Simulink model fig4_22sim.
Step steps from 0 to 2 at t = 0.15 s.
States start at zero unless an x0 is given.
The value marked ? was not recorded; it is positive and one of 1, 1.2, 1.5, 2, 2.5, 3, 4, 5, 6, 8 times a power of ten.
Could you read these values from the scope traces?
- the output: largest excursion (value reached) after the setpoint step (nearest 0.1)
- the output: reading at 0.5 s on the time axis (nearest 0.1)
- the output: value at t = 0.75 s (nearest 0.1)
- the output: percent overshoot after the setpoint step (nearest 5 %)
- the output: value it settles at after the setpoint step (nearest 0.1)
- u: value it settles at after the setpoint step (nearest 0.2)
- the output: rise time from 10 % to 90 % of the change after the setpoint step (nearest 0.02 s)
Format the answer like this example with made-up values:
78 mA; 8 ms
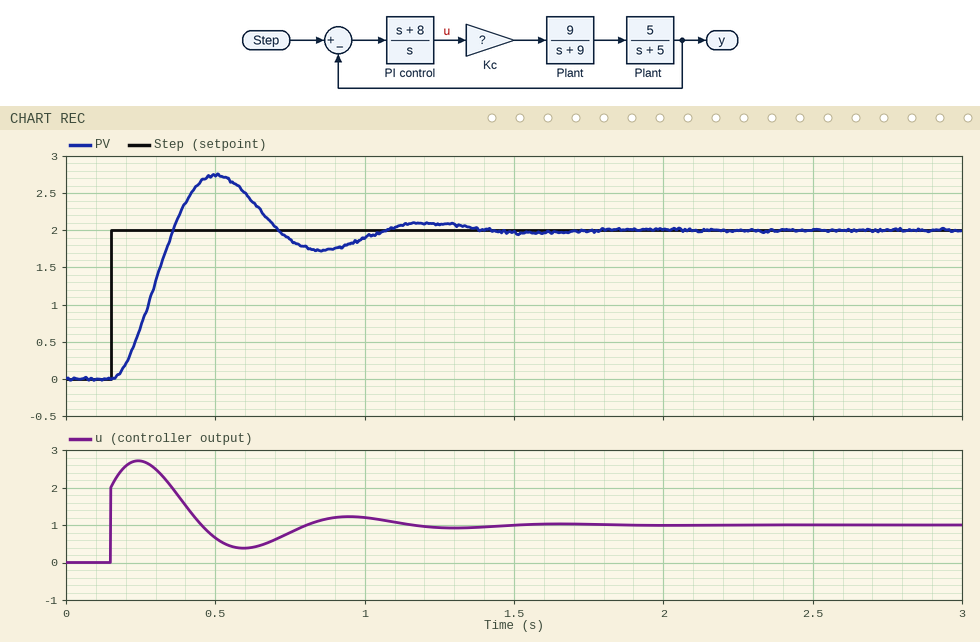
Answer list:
2.7; 2.7; 1.9; 35 %; 2.0; 1.0; 0.14 s
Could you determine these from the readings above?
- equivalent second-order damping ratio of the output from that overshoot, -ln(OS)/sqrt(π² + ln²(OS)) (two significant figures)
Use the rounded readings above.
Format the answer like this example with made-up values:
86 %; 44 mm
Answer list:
0.32
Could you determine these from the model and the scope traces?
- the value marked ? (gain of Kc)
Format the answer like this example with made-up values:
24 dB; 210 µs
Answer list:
2
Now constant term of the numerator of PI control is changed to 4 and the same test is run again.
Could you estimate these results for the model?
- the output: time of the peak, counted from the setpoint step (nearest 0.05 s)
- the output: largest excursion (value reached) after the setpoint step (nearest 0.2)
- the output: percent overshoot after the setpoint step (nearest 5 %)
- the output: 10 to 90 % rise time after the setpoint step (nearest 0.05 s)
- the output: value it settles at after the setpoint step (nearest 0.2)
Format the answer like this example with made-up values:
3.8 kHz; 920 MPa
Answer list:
0.40 s; 2.2; 10 %; 0.20 s; 2.0
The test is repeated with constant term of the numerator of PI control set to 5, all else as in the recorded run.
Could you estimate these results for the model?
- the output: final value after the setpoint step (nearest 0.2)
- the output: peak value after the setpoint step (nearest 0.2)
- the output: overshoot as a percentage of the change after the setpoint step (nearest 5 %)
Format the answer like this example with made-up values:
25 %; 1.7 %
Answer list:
2.0; 2.4; 20 %
